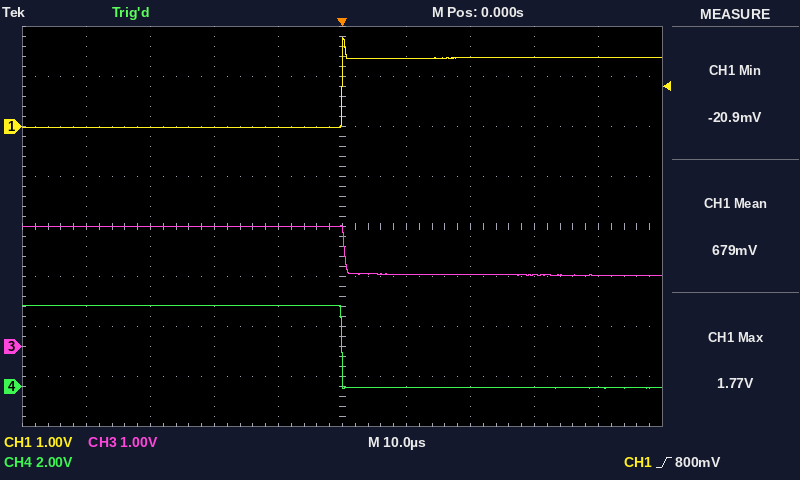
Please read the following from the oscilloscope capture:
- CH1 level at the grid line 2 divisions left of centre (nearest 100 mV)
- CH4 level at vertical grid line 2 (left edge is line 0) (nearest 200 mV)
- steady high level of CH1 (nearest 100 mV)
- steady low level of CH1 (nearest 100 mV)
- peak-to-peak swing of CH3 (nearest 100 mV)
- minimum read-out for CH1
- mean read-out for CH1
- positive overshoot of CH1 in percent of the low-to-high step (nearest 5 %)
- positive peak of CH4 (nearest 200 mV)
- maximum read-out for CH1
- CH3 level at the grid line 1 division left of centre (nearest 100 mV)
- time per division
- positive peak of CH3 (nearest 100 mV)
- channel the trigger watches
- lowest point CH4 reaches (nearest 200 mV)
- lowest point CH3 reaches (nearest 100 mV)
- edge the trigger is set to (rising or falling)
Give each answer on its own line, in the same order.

0.0 V
3.2 V
1.4 V
0.0 V
1.0 V
-20.9 mV
679 mV
30 %
3.2 V
1.77 V
2.4 V
10 µs
2.4 V
CH1
0.0 V
1.4 V
rising
